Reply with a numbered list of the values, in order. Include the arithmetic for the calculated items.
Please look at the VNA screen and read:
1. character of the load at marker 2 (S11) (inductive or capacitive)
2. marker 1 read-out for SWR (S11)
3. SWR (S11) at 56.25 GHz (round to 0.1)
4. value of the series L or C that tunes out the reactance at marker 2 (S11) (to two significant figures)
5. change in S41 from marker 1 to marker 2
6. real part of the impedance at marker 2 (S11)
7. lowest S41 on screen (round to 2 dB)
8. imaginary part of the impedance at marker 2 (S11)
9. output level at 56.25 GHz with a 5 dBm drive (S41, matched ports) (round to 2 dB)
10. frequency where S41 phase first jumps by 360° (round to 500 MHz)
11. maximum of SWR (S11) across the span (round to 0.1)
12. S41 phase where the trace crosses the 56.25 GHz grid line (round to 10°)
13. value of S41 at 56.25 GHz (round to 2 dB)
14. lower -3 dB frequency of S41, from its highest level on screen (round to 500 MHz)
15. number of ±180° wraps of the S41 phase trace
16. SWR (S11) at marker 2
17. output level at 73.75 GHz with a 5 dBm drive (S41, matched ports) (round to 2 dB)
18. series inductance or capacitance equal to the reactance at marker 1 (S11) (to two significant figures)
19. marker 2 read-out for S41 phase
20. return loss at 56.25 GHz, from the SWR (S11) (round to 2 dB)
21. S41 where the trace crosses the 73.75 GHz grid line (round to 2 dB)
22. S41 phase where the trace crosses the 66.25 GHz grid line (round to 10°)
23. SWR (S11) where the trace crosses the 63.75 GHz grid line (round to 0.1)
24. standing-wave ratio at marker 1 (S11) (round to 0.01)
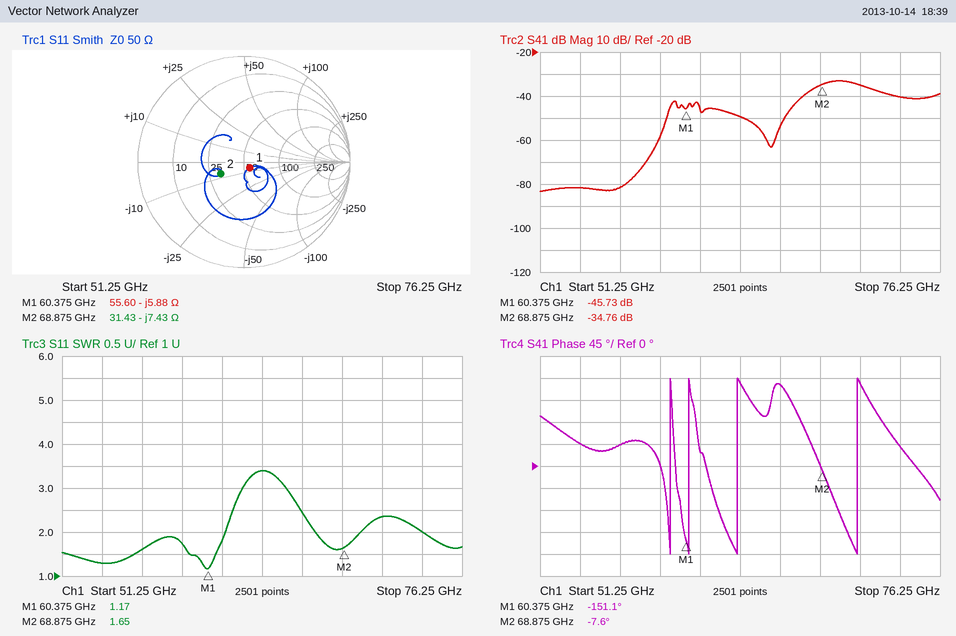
1. capacitive
2. 1.17
3. 1.6
4. L = 7.43 Ω/(2π × 68.875 GHz) ≈ 17 pH
5. -34.76 − (-45.73) = 10.97 dB
6. 31.43 Ω
7. -84 dB
8. -7.43 Ω
9. 5 dBm + (-82 dB) = -76 dBm
10. 59.5 GHz
11. 3.4
12. 40°
13. -82 dB
14. 68.5 GHz
15. 4
16. 1.65
17. 5 dBm + (-40 dB) = -36 dBm
18. C = 1/(2π × 60.375 GHz × 5.88 Ω) ≈ 448 fF, so 450 fF to two significant figures
19. -7.6°
20. −20 log10((1.6 − 1)/(1.6 + 1)) ≈ 12.7 dB, so 12 dB to the nearest 2 dB
21. -40 dB
22. 170°
23. 3.4
24. 1.17
